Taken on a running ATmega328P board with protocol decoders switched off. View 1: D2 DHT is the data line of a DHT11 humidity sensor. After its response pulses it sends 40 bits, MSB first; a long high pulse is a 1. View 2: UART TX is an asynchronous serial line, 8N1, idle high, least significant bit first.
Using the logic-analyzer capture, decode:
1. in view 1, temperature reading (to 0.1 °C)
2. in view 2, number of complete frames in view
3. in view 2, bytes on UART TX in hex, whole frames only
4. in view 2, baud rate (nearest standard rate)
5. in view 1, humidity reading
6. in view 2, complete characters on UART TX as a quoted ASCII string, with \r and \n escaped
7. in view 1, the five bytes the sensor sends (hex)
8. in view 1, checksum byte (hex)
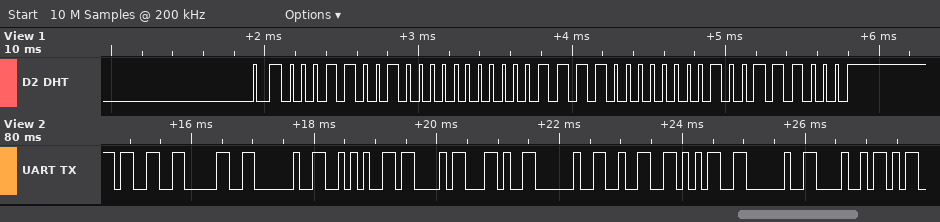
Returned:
30.1 °C
11
33 30 20 2A 43 2C 20 32 35 20 48
9600 baud
25 %
"30 *C, 25 H"
19 00 1E 01 38
0x38
